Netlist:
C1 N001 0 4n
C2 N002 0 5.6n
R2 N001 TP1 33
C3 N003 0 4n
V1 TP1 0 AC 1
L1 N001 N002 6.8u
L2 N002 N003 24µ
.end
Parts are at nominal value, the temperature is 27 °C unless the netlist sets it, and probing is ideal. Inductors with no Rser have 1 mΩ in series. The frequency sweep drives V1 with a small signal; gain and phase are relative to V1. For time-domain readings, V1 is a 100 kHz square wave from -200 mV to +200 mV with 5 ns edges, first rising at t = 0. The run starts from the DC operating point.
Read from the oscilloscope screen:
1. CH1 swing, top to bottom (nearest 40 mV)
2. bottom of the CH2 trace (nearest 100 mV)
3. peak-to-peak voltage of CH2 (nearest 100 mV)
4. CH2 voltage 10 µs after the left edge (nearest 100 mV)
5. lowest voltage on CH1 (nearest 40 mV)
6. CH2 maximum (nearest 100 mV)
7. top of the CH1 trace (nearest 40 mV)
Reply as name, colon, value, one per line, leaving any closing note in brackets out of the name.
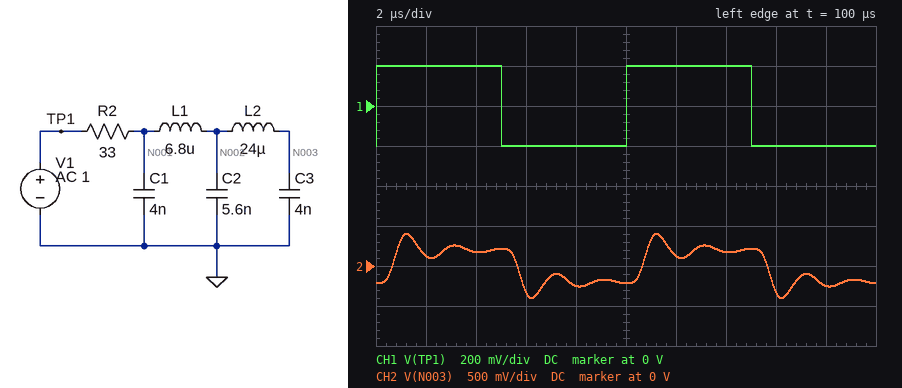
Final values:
CH1 swing, top to bottom: 400 mV
bottom of the CH2 trace: -400 mV
peak-to-peak voltage of CH2: 800 mV
CH2 voltage 10 µs after the left edge: -200 mV
lowest voltage on CH1: -200 mV
CH2 maximum: 400 mV
top of the CH1 trace: 200 mV
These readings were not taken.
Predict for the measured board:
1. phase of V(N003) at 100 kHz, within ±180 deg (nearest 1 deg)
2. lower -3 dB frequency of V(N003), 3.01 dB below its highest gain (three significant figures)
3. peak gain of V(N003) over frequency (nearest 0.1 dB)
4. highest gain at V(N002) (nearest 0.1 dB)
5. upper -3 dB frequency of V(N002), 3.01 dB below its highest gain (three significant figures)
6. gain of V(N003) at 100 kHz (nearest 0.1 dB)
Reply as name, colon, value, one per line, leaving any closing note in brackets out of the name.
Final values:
phase of V(N003) at 100 kHz, within ±180 deg: -16 deg
lower -3 dB frequency of V(N003), 3.01 dB below its highest gain: 391 kHz
peak gain of V(N003) over frequency: 7.6 dB
highest gain at V(N002): 2.5 dB
upper -3 dB frequency of V(N002), 3.01 dB below its highest gain: 1.26 MHz
gain of V(N003) at 100 kHz: 0.2 dB
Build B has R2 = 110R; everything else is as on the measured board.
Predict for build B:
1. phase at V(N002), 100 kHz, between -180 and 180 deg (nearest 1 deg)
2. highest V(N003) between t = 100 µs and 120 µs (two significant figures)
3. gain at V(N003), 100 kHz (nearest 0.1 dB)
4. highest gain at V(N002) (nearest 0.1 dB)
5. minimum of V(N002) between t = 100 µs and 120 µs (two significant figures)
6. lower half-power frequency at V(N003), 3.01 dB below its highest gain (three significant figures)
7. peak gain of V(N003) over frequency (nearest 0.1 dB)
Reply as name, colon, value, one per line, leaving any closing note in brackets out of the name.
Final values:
phase at V(N002), 100 kHz, between -180 and 180 deg: -44 deg
highest V(N003) between t = 100 µs and 120 µs: 210 mV
gain at V(N003), 100 kHz: -2.3 dB
highest gain at V(N002): 0 dB
minimum of V(N002) between t = 100 µs and 120 µs: -190 mV
lower half-power frequency at V(N003), 3.01 dB below its highest gain: 547 kHz
peak gain of V(N003) over frequency: 5.6 dB
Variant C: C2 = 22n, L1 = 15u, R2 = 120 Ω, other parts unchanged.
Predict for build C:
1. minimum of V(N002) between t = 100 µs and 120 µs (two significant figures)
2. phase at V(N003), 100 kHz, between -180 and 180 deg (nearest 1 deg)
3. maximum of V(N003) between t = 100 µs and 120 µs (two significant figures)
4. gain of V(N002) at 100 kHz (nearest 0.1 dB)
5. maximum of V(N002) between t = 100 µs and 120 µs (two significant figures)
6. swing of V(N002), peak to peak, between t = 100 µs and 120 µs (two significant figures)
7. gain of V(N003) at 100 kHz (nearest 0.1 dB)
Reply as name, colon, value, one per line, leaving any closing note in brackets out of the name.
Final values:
minimum of V(N002) between t = 100 µs and 120 µs: -120 mV
phase at V(N003), 100 kHz, between -180 and 180 deg: -69 deg
maximum of V(N003) between t = 100 µs and 120 µs: 160 mV
gain of V(N002) at 100 kHz: -7.5 dB
maximum of V(N002) between t = 100 µs and 120 µs: 120 mV
swing of V(N002), peak to peak, between t = 100 µs and 120 µs: 240 mV
gain of V(N003) at 100 kHz: -7.2 dB
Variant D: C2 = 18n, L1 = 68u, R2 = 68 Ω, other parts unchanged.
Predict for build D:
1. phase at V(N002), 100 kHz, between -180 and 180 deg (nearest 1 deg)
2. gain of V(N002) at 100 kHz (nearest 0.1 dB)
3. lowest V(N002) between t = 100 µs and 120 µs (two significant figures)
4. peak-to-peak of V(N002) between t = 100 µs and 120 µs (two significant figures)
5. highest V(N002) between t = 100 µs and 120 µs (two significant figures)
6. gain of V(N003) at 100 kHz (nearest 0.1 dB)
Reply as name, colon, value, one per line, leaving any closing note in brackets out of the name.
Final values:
phase at V(N002), 100 kHz, between -180 and 180 deg: -68 deg
gain of V(N002) at 100 kHz: -0.8 dB
lowest V(N002) between t = 100 µs and 120 µs: -220 mV
peak-to-peak of V(N002) between t = 100 µs and 120 µs: 440 mV
highest V(N002) between t = 100 µs and 120 µs: 220 mV
gain of V(N003) at 100 kHz: -0.4 dB
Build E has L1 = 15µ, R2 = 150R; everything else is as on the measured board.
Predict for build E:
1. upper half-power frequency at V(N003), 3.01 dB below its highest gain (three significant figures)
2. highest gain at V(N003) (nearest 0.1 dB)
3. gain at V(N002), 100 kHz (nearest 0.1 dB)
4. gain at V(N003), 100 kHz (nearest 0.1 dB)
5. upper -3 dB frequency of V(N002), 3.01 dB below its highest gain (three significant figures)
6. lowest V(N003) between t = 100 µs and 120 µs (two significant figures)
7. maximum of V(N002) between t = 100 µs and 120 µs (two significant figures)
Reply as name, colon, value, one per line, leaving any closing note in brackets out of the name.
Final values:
upper half-power frequency at V(N003), 3.01 dB below its highest gain: 601 kHz
highest gain at V(N003): 2.7 dB
gain at V(N002), 100 kHz: -4.0 dB
gain at V(N003), 100 kHz: -3.7 dB
upper -3 dB frequency of V(N002), 3.01 dB below its highest gain: 955 kHz
lowest V(N003) between t = 100 µs and 120 µs: -190 mV
maximum of V(N002) between t = 100 µs and 120 µs: 180 mV
